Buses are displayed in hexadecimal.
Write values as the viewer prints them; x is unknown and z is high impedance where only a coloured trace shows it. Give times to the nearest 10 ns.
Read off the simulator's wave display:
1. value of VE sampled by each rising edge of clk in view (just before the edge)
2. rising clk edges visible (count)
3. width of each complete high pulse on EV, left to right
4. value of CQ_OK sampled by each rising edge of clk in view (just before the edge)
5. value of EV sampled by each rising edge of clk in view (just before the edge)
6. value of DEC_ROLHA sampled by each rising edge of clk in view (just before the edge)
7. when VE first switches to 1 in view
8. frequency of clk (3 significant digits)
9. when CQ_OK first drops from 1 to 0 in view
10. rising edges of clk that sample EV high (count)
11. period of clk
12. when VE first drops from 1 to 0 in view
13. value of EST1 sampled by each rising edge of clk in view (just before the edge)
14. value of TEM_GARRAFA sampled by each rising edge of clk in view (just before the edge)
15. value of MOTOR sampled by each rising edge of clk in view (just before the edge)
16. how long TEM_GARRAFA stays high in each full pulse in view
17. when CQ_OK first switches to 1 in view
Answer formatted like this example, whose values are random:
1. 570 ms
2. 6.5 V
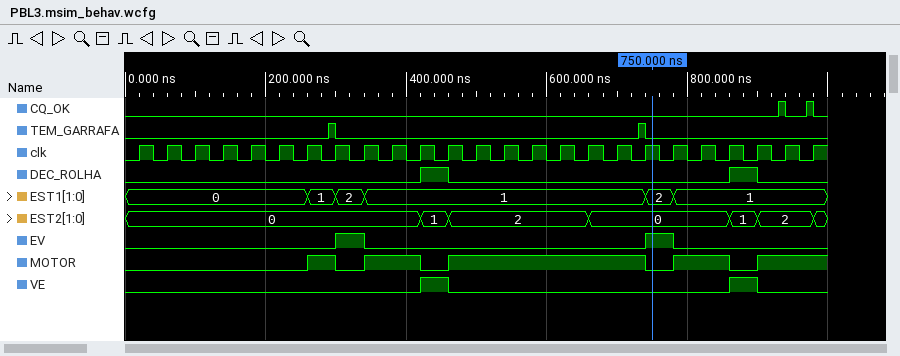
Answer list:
1. 0 0 0 0 0 0 0 0 0 0 0 1 0 0 0 0 0 0 0 0 0 0 1 0 0
2. 25
3. 40 ns, 40 ns
4. 0 0 0 0 0 0 0 0 0 0 0 0 0 0 0 0 0 0 0 0 0 0 0 1 1
5. 0 0 0 0 0 0 0 0 1 0 0 0 0 0 0 0 0 0 0 1 0 0 0 0 0
6. 0 0 0 0 0 0 0 0 0 0 0 1 0 0 0 0 0 0 0 0 0 0 1 0 0
7. 420 ns
8. 25.0 MHz
9. 940 ns
10. 2
11. 40 ns
12. 460 ns
13. 0, 0, 0, 0, 0, 0, 0, 1, 2, 1, 1, 1, 1, 1, 1, 1, 1, 1, 1, 2, 1, 1, 1, 1, 1
14. 0 0 0 0 0 0 0 1 0 0 0 0 0 0 0 0 0 0 1 0 0 0 0 0 0
15. 0 0 0 0 0 0 0 1 0 1 1 0 1 1 1 1 1 1 1 0 1 1 0 1 1
16. 10 ns, 10 ns
17. 930 ns
